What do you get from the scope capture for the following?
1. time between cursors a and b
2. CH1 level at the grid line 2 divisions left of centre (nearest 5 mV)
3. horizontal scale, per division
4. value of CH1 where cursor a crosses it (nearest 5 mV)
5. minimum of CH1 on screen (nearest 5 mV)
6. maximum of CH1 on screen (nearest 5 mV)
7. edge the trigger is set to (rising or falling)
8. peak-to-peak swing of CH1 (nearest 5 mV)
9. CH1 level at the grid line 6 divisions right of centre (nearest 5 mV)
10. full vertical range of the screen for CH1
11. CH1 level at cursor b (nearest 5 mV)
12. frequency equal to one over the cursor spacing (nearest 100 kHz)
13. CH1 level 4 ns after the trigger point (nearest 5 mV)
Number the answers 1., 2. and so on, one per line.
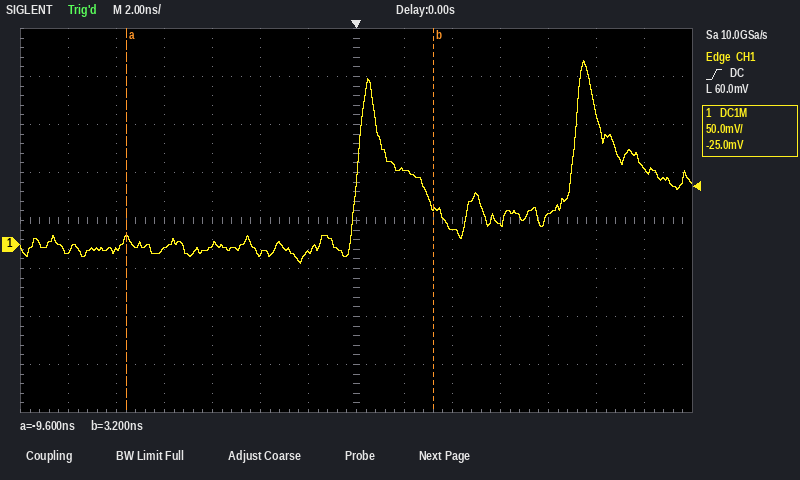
1. 12.8 ns
2. -10 mV
3. 2 ns
4. 5 mV
5. -20 mV
6. 190 mV
7. rising
8. 210 mV
9. 80 mV
10. 400 mV
11. 40 mV
12. 78.1 MHz
13. 15 mV
